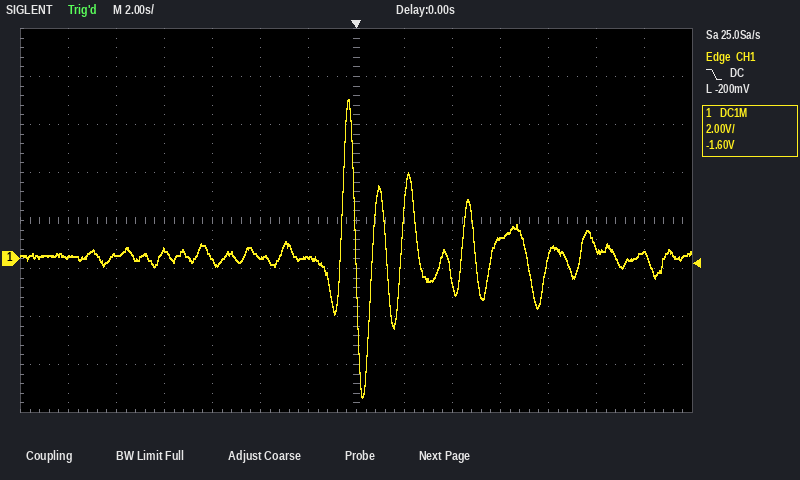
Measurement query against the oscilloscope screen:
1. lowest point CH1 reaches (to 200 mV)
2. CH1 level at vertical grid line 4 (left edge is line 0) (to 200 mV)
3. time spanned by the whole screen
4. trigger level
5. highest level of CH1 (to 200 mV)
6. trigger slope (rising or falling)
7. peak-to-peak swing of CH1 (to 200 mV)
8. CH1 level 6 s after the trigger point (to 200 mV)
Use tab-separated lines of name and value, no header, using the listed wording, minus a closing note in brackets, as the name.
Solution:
lowest point CH1 reaches	-5.8 V
CH1 level at vertical grid line 4 (left edge is line 0)	0.0 V
time spanned by the whole screen	28 s
trigger level	-200 mV
highest level of CH1	6.6 V
trigger slope	falling
peak-to-peak swing of CH1	12.4 V
CH1 level 6 s after the trigger point	800 mV
